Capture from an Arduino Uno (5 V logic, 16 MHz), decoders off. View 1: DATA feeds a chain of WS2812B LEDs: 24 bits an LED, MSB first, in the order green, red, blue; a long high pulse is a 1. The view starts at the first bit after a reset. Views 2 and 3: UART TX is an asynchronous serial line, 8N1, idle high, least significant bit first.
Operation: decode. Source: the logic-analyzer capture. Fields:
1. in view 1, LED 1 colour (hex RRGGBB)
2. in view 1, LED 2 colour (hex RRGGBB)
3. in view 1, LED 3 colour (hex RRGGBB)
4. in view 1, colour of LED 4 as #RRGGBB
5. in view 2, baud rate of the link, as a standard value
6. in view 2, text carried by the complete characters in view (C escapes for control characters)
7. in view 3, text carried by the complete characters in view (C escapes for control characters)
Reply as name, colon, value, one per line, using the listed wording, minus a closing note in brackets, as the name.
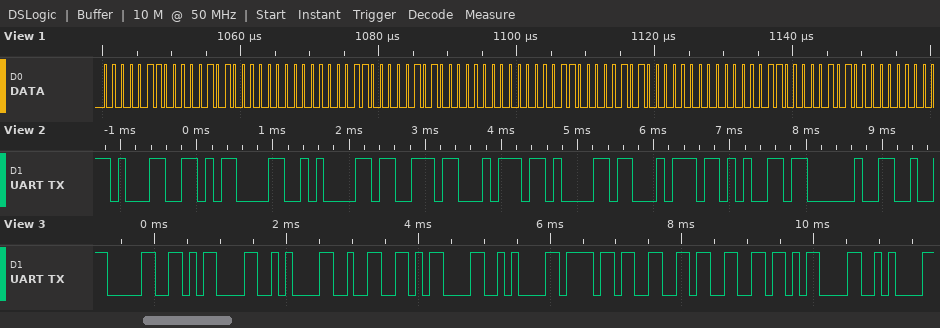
in view 1, LED 1 colour: #0A0600
in view 1, LED 2 colour: #0A0600
in view 1, LED 3 colour: #0A0600
in view 1, colour of LED 4 as #RRGGBB: #0A0600
in view 2, baud rate of the link, as a standard value: 9600 baud
in view 2, text carried by the complete characters in view: "1\r\nstate "
in view 3, text carried by the complete characters in view: "0\r\n2\r\noff\r\n"
